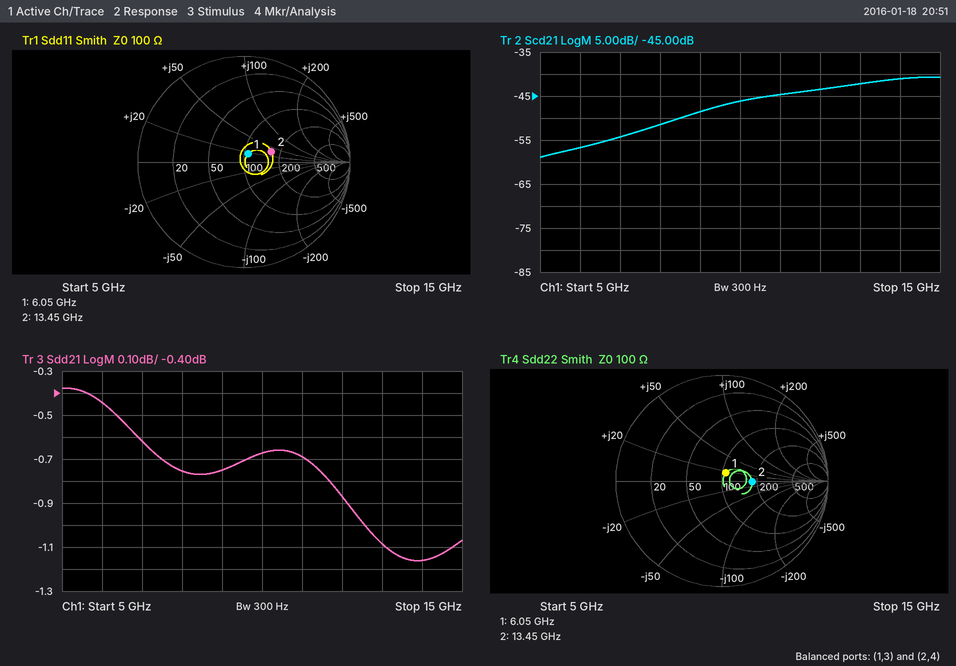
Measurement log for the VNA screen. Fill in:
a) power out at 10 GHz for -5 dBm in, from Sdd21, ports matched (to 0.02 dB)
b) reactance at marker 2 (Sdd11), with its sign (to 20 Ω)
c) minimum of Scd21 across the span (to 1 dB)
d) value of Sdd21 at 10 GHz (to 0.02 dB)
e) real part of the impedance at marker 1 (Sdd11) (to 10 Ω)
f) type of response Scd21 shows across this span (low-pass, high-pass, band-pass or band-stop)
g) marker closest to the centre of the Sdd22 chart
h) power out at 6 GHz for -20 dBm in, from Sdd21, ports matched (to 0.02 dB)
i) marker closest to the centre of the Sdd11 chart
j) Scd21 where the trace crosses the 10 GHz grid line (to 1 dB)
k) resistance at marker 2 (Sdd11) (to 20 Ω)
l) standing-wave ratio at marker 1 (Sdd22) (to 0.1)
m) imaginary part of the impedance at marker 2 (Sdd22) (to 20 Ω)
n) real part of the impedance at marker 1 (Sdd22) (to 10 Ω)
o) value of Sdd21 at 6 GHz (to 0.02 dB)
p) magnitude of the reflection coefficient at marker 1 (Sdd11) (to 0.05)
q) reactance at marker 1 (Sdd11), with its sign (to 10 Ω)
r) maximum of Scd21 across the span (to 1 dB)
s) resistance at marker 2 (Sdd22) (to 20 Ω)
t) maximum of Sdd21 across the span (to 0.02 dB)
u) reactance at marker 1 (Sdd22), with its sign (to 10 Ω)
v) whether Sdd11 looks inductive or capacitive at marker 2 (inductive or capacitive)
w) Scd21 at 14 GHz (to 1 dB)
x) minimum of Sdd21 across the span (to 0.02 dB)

-5.68 dBm
+40 Ω
-59 dB
-0.68 dB
110 Ω
high-pass
marker 1
-20.44 dBm
marker 1
-46 dB
160 Ω
1.2
0 Ω
110 Ω
-0.44 dB
0.10
+20 Ω
-41 dB
180 Ω
-0.38 dB
+20 Ω
inductive
-41 dB
-1.16 dB
